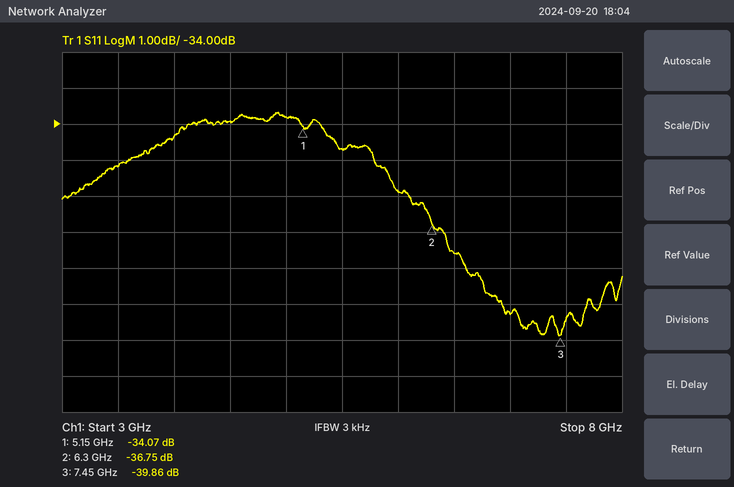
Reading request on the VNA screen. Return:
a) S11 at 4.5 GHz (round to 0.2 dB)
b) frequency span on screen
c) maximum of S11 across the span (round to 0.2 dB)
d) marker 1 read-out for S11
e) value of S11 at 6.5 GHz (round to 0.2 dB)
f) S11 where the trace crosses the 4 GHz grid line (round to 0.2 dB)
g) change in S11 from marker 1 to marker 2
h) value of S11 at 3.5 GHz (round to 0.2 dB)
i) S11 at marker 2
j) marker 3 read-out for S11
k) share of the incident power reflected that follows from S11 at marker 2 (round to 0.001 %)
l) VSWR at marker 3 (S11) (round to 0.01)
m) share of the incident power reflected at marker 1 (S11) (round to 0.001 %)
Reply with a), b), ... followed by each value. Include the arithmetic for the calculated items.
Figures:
a) -34.0 dB
b) 5 GHz
c) -33.6 dB
d) -34.07 dB
e) -37.6 dB
f) -34.4 dB
g) -36.75 − (-34.07) = -2.68 dB
h) -35.2 dB
i) -36.75 dB
j) -39.86 dB
k) 10^(-36.75/10) ≈ 0.021 %
l) (1 + 0.0102)/(1 − 0.0102) ≈ 1.02
m) 10^(-34.07/10) ≈ 0.039 %
